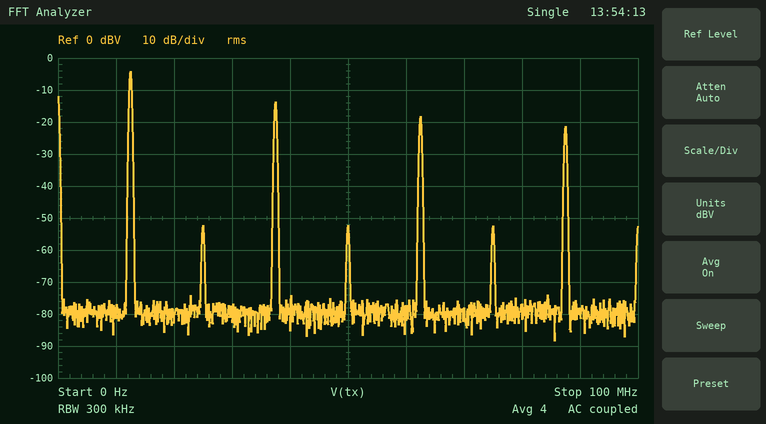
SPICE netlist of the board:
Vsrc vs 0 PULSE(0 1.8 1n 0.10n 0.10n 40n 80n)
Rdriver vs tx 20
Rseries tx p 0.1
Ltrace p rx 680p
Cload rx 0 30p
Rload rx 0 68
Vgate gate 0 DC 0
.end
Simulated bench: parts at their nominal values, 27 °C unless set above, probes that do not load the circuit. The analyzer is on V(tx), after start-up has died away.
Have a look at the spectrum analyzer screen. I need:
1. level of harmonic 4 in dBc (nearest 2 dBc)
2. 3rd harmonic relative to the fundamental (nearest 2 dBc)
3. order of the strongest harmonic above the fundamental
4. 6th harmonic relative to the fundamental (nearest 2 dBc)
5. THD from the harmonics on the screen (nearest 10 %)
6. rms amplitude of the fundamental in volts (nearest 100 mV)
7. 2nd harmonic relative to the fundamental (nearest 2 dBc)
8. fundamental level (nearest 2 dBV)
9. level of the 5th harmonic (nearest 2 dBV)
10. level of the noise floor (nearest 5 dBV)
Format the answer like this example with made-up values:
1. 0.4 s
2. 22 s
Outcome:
1. -48 dBc
2. -10 dBc
3. 3
4. -48 dBc
5. 40 %
6. 600 mV
7. -48 dBc
8. -4 dBV
9. -18 dBV
10. -80 dBV
